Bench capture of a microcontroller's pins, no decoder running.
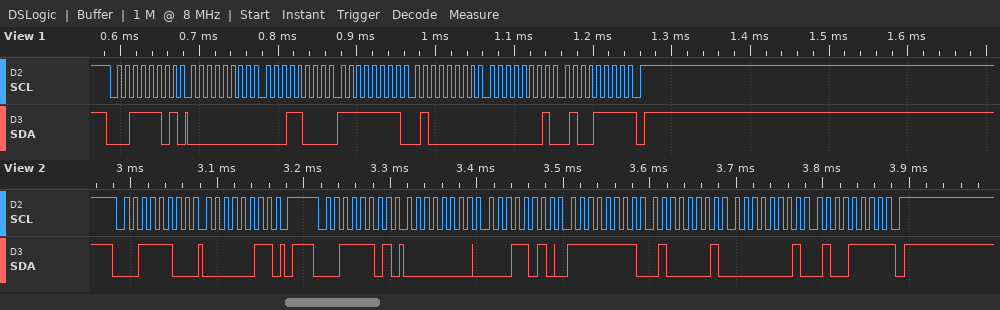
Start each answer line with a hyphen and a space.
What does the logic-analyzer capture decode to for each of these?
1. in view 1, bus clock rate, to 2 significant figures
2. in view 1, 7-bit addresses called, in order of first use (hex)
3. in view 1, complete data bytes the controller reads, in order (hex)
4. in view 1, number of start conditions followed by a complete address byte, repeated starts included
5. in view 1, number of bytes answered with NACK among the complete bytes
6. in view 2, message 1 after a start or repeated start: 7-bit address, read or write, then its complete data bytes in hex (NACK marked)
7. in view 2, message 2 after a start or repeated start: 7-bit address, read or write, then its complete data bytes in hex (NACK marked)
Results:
- 100 kHz
- 0x1E
- 00 18 FF 40 01 4F
- 1
- 1
- 0x1E write: 03
- 0x1E read: 00 1A FF 41 01 4F NACK
